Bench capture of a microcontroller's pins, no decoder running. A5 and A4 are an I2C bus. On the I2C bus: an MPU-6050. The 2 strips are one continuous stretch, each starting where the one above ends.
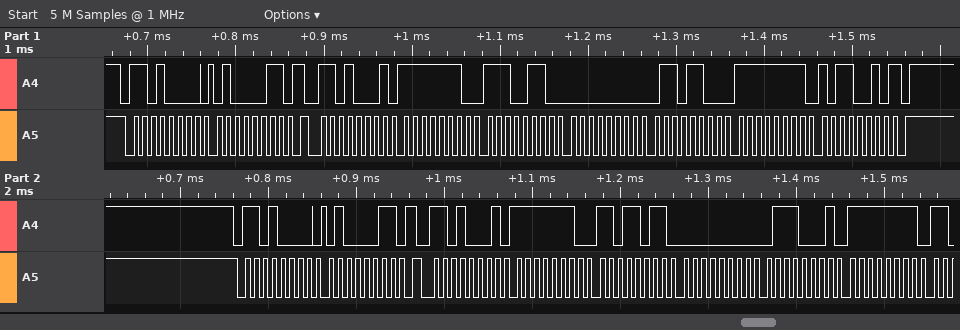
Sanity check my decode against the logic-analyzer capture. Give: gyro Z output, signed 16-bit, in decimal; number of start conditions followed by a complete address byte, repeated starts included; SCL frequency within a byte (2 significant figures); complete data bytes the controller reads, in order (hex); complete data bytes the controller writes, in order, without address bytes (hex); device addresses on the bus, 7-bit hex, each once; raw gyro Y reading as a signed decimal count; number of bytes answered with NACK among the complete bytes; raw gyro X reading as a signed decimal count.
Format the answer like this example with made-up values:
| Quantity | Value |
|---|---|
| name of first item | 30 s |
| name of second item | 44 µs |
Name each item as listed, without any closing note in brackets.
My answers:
| Quantity | Value |
|---|---|
| gyro Z output, signed 16-bit, in decimal | -78 |
| number of start conditions followed by a complete address byte, repeated starts included | 4 |
| SCL frequency within a byte | 100 kHz |
| complete data bytes the controller reads, in order | FE E6 00 6C FF B2 FE DB 00 71 FF |
| complete data bytes the controller writes, in order, without address bytes | 43 43 |
| device addresses on the bus, 7-bit hex, each once | 0x68 |
| raw gyro Y reading as a signed decimal count | 108 |
| number of bytes answered with NACK among the complete bytes | 1 |
| raw gyro X reading as a signed decimal count | -282 |
